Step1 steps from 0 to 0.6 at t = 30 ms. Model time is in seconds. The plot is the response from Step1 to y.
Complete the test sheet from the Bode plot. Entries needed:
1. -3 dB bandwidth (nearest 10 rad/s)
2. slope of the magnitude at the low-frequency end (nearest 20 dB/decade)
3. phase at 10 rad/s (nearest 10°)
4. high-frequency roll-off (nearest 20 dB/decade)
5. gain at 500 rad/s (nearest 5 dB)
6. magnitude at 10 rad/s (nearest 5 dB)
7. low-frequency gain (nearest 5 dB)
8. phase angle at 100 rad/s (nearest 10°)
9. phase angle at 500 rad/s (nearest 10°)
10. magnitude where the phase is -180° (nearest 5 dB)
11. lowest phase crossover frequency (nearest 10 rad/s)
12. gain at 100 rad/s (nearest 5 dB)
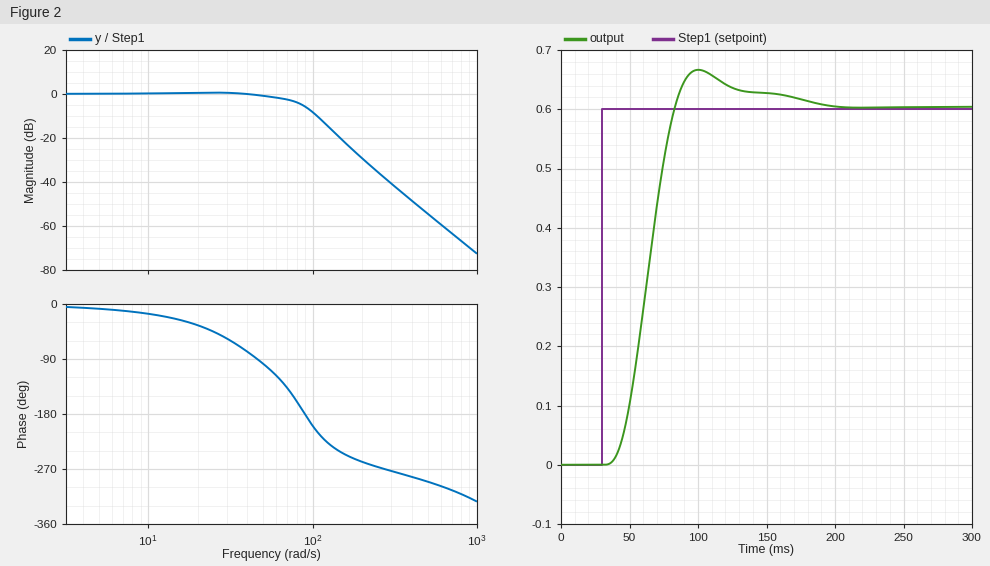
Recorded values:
70 rad/s
0 dB/decade
-20°
-60 dB/decade
-55 dB
0 dB
0 dB
-200°
-290°
-5 dB
90 rad/s
-10 dB
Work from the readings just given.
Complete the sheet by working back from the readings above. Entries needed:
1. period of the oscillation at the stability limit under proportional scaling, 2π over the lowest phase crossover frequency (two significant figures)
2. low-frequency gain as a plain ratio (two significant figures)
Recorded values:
0.070 s
1.0
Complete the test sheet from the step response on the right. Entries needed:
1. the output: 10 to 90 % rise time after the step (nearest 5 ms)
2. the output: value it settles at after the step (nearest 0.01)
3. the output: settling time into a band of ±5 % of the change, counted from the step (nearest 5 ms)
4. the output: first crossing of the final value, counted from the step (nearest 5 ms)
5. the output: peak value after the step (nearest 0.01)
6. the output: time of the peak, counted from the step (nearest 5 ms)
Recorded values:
30 ms
0.60
100 ms
55 ms
0.67
70 ms
